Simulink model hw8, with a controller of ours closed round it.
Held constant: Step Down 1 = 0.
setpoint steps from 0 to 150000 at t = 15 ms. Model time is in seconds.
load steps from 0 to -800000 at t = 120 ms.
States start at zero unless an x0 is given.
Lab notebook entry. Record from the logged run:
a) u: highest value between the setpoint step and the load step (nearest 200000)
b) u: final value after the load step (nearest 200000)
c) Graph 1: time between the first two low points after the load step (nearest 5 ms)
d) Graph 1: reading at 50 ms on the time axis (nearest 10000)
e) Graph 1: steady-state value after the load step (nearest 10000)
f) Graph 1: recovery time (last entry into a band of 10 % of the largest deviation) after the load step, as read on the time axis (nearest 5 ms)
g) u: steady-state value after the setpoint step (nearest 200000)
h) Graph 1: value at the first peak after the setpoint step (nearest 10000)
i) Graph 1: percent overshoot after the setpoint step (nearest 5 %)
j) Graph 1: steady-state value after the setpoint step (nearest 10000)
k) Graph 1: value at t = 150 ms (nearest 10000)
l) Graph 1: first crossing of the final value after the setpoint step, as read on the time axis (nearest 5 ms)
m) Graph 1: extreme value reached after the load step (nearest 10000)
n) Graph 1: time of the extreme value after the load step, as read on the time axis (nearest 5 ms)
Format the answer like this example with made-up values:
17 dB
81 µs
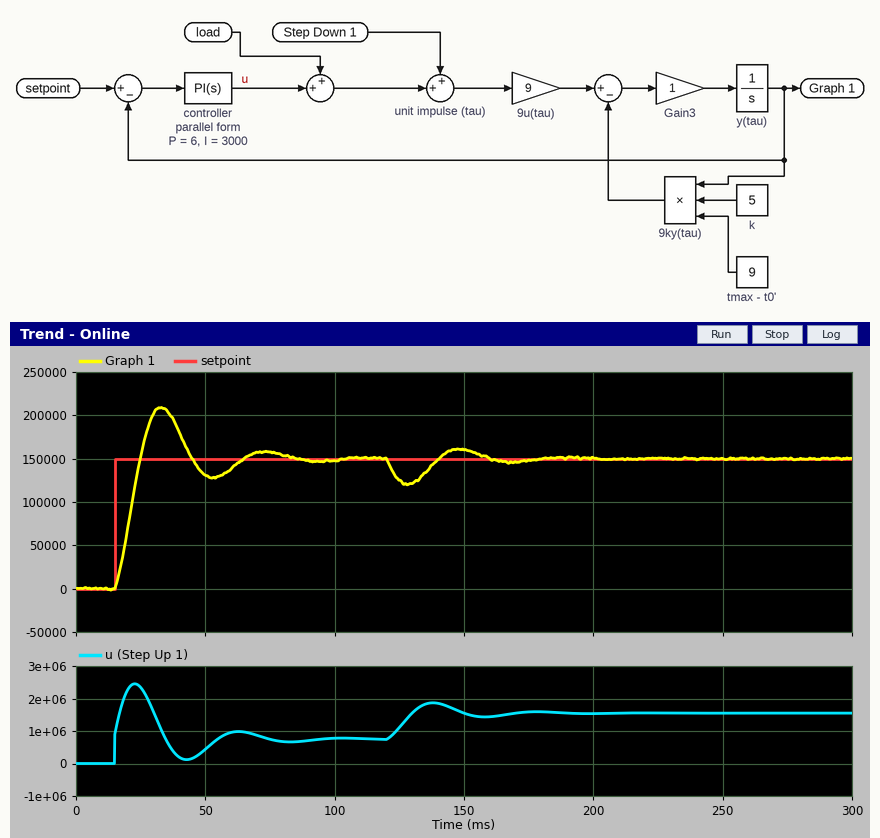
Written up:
2400000
1600000
40 ms
130000
150000
175 ms
800000
210000
40 %
150000
160000
25 ms
120000
130 ms
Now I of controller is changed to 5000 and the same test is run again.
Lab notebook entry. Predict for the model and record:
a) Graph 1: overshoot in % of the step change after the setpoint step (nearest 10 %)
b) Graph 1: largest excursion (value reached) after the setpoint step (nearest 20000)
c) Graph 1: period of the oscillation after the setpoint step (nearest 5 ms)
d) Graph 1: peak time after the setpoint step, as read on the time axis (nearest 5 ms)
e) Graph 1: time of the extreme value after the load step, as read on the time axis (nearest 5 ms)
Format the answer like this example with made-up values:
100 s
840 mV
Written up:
50 %
220000
30 ms
30 ms
125 ms
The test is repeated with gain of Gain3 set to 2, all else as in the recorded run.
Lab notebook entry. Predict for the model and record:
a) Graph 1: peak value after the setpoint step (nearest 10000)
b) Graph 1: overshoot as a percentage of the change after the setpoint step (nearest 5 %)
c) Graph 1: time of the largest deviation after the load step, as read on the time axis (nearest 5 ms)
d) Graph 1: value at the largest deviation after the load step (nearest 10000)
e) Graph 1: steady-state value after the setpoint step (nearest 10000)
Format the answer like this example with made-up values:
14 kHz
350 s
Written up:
190000
25 %
125 ms
110000
150000
